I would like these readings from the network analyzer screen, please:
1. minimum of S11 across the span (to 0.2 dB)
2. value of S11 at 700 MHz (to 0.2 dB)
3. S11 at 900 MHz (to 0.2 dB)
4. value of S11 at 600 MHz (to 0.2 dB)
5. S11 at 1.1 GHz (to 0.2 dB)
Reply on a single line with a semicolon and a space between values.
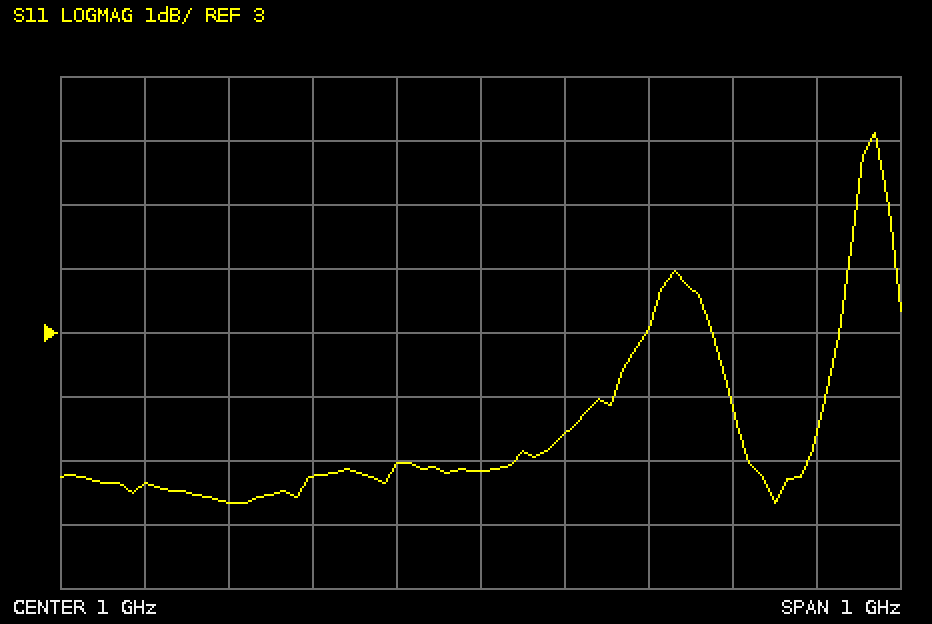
0.4 dB; 0.4 dB; 1.0 dB; 0.6 dB; 1.4 dB
